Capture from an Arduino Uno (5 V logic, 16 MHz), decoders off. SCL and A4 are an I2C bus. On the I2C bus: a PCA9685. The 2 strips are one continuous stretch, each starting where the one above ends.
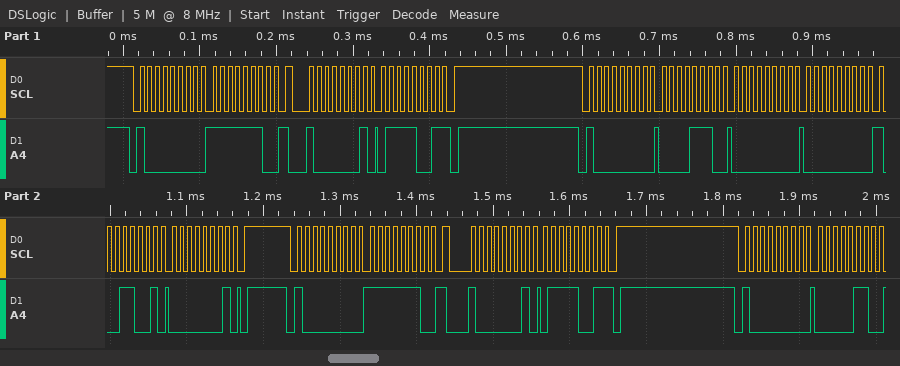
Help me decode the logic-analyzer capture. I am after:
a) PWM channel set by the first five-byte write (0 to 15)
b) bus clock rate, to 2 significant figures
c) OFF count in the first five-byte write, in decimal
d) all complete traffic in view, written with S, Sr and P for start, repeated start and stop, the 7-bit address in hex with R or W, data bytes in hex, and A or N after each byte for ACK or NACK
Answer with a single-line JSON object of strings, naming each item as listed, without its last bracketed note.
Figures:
{"PWM channel set by the first five-byte write": "2", "bus clock rate, to 2 significant figures": "100 kHz", "OFF count in the first five-byte write, in decimal": "409", "all complete traffic in view, written with S, Sr and P for start, repeated start and stop, the 7-bit address in hex with R or W, data bytes in hex, and A or N after each byte for ACK or NACK": "S 40W A FE A Sr 40R A 79 N P S 40W A 0E A 00 A 00 A 99 A 01 A P S 40W A FE A Sr 40R A 79 N P S 40W A 06 A"}
